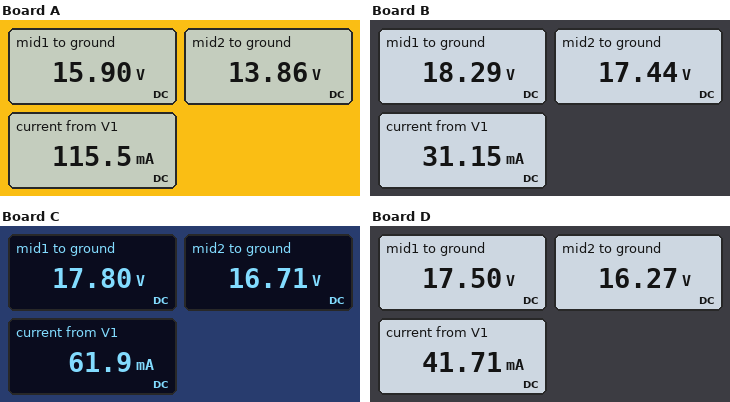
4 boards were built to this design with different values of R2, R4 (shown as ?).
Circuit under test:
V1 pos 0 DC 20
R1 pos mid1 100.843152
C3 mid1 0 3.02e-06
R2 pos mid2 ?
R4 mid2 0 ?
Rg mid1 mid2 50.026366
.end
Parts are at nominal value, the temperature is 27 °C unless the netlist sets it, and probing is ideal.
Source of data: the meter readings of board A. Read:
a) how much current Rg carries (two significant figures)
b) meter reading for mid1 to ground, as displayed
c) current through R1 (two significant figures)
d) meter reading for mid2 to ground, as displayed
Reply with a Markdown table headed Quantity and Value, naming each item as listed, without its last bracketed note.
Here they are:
| Quantity | Value |
|---|---|
| how much current Rg carries | 41 mA |
| meter reading for mid1 to ground, as displayed | 15.90 V |
| current through R1 | 41 mA |
| meter reading for mid2 to ground, as displayed | 13.86 V |
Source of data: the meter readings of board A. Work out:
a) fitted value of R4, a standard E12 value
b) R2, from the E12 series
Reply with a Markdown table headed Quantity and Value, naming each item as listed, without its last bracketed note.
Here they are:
| Quantity | Value |
|---|---|
| fitted value of R4, a standard E12 value | 120 Ω |
| R2, from the E12 series | 82 Ω |
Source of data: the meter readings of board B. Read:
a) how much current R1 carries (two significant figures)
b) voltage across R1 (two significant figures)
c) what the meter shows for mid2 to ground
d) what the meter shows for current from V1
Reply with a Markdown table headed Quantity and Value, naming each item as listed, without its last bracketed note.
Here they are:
| Quantity | Value |
|---|---|
| how much current R1 carries | 17 mA |
| voltage across R1 | 1.7 V |
| what the meter shows for mid2 to ground | 17.44 V |
| what the meter shows for current from V1 | 31.15 mA |
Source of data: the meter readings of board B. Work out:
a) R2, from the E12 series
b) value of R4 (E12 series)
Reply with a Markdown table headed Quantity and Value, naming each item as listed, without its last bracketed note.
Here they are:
| Quantity | Value |
|---|---|
| R2, from the E12 series | 180 Ω |
| value of R4 | 560 Ω |
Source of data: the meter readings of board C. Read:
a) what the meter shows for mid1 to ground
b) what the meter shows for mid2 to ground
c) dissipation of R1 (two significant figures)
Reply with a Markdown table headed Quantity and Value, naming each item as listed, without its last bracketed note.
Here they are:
| Quantity | Value |
|---|---|
| what the meter shows for mid1 to ground | 17.80 V |
| what the meter shows for mid2 to ground | 16.71 V |
| dissipation of R1 | 48 mW |
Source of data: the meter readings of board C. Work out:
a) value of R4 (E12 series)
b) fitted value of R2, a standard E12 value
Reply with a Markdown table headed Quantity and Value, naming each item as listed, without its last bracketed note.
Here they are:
| Quantity | Value |
|---|---|
| value of R4 | 270 Ω |
| fitted value of R2, a standard E12 value | 82 Ω |
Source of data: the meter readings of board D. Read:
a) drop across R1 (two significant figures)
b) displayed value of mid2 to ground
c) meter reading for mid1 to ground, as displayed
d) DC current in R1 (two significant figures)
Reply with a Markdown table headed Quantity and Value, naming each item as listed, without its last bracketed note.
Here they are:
| Quantity | Value |
|---|---|
| drop across R1 | 2.5 V |
| displayed value of mid2 to ground | 16.27 V |
| meter reading for mid1 to ground, as displayed | 17.50 V |
| DC current in R1 | 25 mA |
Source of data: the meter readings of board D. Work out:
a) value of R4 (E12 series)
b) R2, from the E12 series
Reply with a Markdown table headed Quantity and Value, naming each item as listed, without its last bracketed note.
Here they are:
| Quantity | Value |
|---|---|
| value of R4 | 390 Ω |
| R2, from the E12 series | 220 Ω |
